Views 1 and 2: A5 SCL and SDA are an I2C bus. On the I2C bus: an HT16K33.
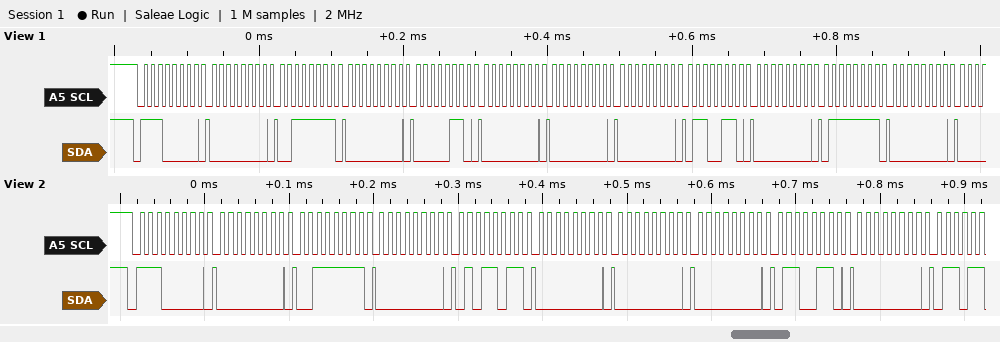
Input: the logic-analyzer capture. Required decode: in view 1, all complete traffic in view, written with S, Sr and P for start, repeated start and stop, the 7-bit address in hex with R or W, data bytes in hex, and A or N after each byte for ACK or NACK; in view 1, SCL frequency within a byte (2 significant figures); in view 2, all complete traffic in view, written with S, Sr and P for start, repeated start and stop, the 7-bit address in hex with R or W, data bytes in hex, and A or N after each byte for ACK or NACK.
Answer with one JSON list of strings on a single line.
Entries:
["S 70W A 00 A 3F A 00 A 06 A 00 A 00 A 00 A 66 A 00 A 7F A 00 A", "100 kHz", "S 70W A 00 A 3F A 00 A 5B A 00 A 00 A 00 A 66 A 00 A"]
